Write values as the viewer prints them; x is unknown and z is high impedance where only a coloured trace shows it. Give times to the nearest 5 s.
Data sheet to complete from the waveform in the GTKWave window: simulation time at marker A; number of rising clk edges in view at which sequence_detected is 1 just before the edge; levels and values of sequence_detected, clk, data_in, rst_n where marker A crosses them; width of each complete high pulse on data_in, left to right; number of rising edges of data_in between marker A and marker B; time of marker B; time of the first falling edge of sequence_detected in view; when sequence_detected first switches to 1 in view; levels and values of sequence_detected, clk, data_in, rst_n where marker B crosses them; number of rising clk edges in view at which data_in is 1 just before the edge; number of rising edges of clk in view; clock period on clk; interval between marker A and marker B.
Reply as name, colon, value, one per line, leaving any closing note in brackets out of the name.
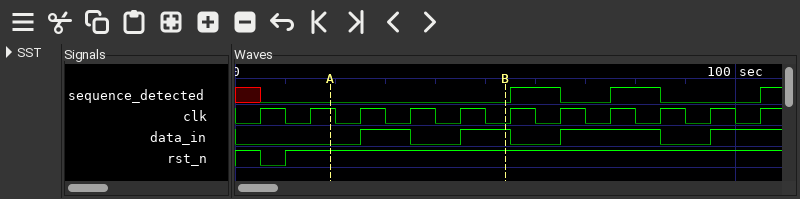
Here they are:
simulation time at marker A: 20 s
number of rising clk edges in view at which sequence_detected is 1 just before the edge: 2
levels and values of sequence_detected, clk, data_in, rst_n where marker A crosses them: sequence_detected=0, clk=1, data_in=0, rst_n=1
width of each complete high pulse on data_in, left to right: 10 s, 10 s, 20 s
number of rising edges of data_in between marker A and marker B: 2
time of marker B: 55 s
time of the first falling edge of sequence_detected in view: 65 s
when sequence_detected first switches to 1 in view: 55 s
levels and values of sequence_detected, clk, data_in, rst_n where marker B crosses them: sequence_detected=0, clk=0, data_in=1, rst_n=1
number of rising clk edges in view at which data_in is 1 just before the edge: 5
number of rising edges of clk in view: 11
clock period on clk: 10 s
interval between marker A and marker B: 35 s
